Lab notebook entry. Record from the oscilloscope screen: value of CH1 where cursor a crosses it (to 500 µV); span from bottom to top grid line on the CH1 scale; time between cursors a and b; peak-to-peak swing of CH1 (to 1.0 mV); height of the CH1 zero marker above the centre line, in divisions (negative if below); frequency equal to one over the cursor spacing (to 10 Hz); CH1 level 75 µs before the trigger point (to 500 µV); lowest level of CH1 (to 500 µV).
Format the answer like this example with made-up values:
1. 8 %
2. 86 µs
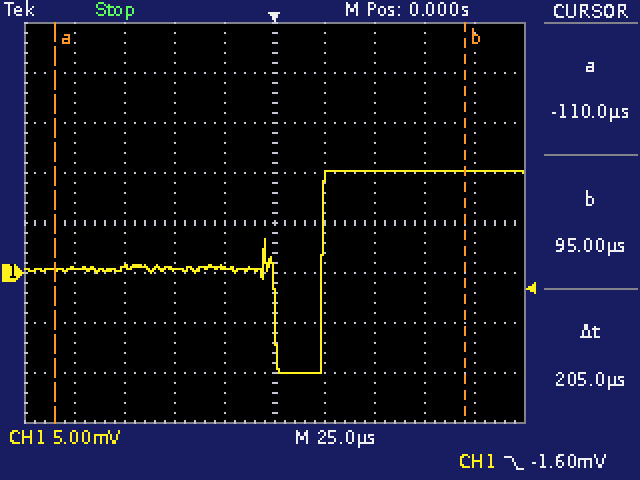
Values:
1. 500 µV
2. 40 mV
3. 205 µs
4. 20.0 mV
5. -1.0 div
6. 4.88 kHz
7. 500 µV
8. -10.0 mV
